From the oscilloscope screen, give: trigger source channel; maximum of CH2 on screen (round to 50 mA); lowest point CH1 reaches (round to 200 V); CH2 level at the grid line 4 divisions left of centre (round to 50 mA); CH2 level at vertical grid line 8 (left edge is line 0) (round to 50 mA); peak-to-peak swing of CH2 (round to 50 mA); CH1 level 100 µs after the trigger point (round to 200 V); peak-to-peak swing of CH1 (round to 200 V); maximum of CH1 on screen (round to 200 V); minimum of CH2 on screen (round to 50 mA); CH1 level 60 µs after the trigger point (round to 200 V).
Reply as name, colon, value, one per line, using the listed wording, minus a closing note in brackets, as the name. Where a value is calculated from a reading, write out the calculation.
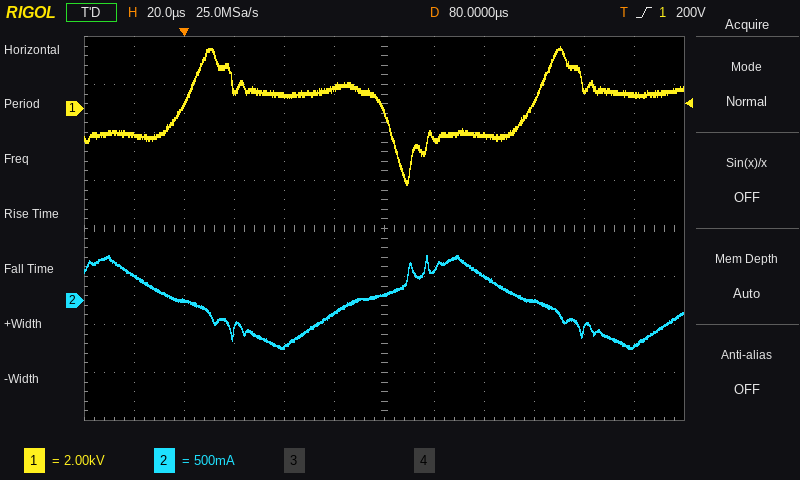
trigger source channel: CH1
maximum of CH2 on screen: 450 mA
lowest point CH1 reaches: -3.2 kV
CH2 level at the grid line 4 divisions left of centre: 0 mA
CH2 level at vertical grid line 8 (left edge is line 0): 250 mA
peak-to-peak swing of CH2: 450 mA − (-500 mA) = 950 mA
CH1 level 100 µs after the trigger point: -1.2 kV
peak-to-peak swing of CH1: 2.6 kV − (-3.2 kV) = 5.8 kV
maximum of CH1 on screen: 2.6 kV
minimum of CH2 on screen: -500 mA
CH1 level 60 µs after the trigger point: 800 V
